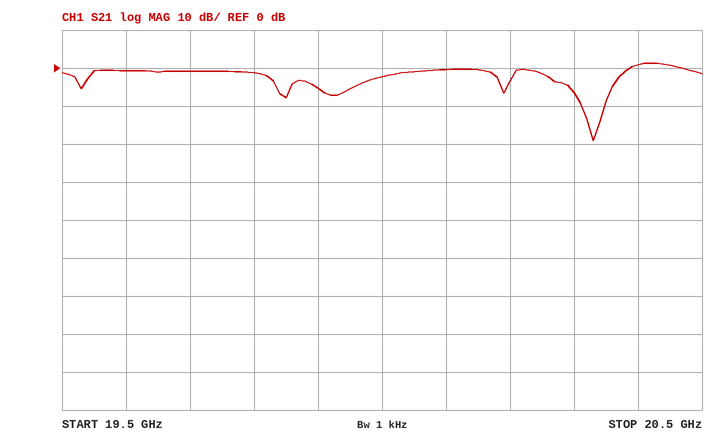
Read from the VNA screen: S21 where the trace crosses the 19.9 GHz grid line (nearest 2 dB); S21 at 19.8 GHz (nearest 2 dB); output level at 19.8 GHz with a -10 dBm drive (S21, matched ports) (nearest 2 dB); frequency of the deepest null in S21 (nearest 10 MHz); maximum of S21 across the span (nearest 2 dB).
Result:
-6 dB
-2 dB
-12 dBm
20.33 GHz
2 dB
